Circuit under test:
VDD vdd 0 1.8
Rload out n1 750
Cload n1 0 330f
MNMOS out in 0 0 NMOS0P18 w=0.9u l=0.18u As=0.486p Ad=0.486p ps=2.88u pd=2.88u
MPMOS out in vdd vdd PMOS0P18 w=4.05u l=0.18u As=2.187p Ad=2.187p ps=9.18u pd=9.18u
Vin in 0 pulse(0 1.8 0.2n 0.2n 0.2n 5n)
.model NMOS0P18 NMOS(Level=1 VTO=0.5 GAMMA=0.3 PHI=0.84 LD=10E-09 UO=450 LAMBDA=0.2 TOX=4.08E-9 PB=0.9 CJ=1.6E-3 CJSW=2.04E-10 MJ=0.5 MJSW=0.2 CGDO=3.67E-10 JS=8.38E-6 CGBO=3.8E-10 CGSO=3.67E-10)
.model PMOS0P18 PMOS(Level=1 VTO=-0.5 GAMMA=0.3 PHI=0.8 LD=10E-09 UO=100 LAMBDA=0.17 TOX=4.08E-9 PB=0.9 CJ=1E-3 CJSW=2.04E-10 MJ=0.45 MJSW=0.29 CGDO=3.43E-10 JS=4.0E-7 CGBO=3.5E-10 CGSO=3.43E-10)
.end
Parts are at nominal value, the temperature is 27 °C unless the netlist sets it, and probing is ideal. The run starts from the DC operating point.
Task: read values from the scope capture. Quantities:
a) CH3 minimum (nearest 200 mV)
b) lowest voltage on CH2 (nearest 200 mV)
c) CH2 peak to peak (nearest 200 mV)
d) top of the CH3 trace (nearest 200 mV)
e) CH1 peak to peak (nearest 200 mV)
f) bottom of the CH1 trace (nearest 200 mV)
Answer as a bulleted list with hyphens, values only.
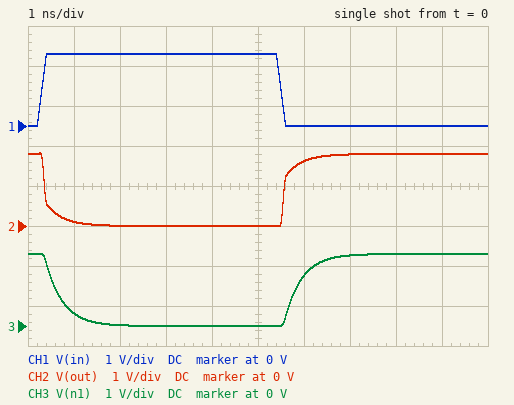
- 0 V
- 0 V
- 1.8 V
- 1.8 V
- 1.8 V
- 0 V
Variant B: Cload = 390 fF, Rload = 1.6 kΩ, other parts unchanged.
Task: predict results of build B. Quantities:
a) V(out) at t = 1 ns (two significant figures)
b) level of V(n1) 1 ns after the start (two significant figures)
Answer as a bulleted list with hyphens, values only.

- 140 mV
- 760 mV
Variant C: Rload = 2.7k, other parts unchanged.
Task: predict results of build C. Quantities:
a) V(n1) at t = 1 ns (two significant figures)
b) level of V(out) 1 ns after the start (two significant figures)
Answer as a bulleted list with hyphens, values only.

- 930 mV
- 110 mV
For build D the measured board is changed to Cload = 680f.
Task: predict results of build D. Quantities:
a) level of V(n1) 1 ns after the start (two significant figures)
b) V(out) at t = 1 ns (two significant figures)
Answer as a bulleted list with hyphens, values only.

- 780 mV
- 260 mV
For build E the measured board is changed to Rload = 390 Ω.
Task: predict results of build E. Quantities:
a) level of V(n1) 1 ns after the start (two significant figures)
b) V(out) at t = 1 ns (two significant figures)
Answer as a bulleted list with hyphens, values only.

- 150 mV
- 71 mV
